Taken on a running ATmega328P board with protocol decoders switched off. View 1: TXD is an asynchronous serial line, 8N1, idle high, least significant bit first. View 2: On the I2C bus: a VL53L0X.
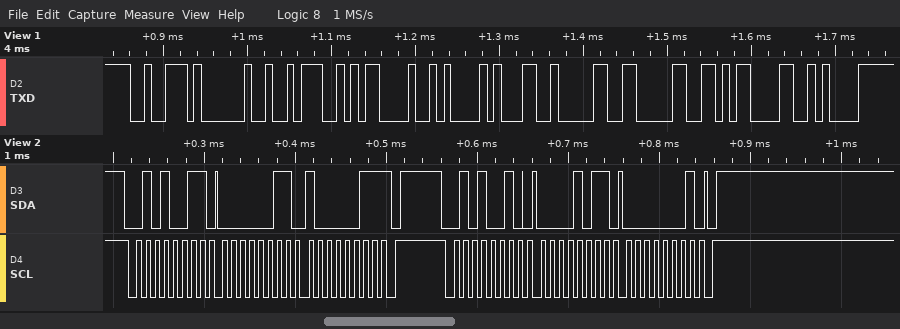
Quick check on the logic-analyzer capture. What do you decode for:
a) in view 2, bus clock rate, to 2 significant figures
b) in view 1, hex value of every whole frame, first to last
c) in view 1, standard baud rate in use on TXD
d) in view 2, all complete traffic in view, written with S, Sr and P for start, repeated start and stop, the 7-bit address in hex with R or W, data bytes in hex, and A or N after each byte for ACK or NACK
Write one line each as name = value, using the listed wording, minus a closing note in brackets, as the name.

in view 2, bus clock rate, to 2 significant figures = 100 kHz
in view 1, hex value of every whole frame, first to last = 72 20 3A 0D 0A 31 30 30 0D 0A
in view 1, standard baud rate in use on TXD = 115200 baud
in view 2, all complete traffic in view, written with S, Sr and P for start, repeated start and stop, the 7-bit address in hex with R or W, data bytes in hex, and A or N after each byte for ACK or NACK = S 29R A 03 A 83 N P S 29W A 0B A 01 A P
